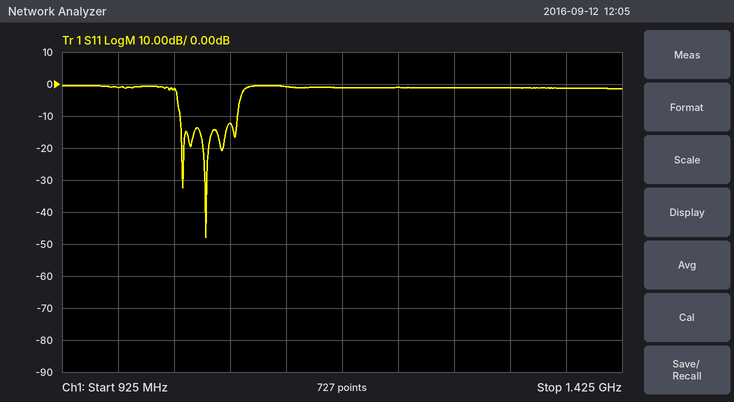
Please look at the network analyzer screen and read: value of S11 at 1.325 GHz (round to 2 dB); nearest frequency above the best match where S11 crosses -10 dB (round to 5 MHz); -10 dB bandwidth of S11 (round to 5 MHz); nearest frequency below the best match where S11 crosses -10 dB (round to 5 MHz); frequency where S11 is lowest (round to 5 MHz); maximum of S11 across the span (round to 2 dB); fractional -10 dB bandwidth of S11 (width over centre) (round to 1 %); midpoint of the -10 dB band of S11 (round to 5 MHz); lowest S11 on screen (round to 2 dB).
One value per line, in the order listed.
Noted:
-2 dB
1.080 GHz
50 MHz
1.030 GHz
1.055 GHz
0 dB
5 %
1.055 GHz
-48 dB
